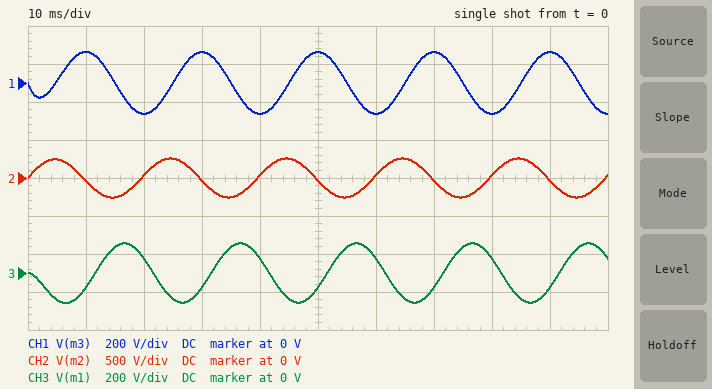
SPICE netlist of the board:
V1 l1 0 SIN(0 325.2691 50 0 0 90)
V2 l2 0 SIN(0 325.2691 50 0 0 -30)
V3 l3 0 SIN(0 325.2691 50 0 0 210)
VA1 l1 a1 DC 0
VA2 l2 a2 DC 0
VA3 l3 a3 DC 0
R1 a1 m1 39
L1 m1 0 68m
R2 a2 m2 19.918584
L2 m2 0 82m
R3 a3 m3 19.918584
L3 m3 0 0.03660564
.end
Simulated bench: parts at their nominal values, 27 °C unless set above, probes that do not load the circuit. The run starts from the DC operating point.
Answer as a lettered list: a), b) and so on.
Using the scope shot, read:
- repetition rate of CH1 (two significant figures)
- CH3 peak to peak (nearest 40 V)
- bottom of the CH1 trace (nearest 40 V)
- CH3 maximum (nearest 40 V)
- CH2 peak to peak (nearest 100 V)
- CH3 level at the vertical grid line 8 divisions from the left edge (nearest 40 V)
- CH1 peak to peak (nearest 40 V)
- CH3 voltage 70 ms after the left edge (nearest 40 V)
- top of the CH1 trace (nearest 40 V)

a) 50 Hz
b) 320 V
c) -160 V
d) 160 V
e) 500 V
f) 80 V
g) 320 V
h) -80 V
i) 160 V
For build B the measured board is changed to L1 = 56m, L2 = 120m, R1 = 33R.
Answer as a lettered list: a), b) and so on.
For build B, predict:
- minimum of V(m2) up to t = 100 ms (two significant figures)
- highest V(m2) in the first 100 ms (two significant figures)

a) -290 V
b) 290 V
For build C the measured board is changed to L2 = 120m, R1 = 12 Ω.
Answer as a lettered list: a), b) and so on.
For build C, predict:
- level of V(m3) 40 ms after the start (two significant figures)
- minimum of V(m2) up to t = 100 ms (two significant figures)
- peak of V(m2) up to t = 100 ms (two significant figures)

a) -160 V
b) -290 V
c) 290 V
